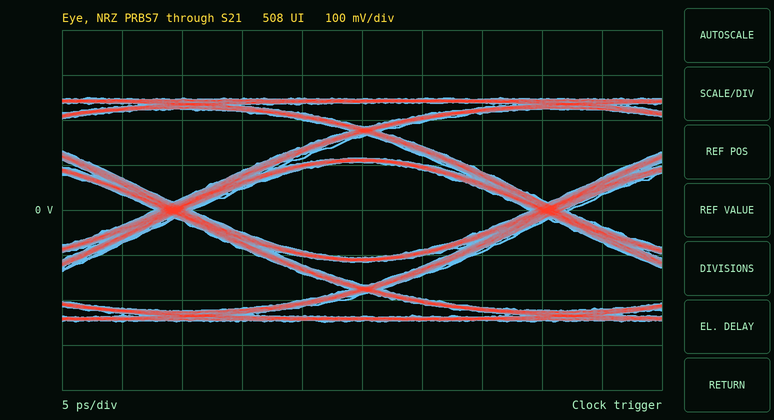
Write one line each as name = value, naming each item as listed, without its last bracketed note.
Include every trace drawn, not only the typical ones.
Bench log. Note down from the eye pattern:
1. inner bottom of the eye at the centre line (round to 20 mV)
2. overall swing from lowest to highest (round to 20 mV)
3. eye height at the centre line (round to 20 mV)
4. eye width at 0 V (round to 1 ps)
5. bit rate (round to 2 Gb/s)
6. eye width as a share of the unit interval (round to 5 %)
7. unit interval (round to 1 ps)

inner bottom of the eye at the centre line = -100 mV
overall swing from lowest to highest = 500 mV
eye height at the centre line = 220 mV
eye width at 0 V = 28 ps
bit rate = 32 Gb/s
eye width as a share of the unit interval = 90 %
unit interval = 31 ps
